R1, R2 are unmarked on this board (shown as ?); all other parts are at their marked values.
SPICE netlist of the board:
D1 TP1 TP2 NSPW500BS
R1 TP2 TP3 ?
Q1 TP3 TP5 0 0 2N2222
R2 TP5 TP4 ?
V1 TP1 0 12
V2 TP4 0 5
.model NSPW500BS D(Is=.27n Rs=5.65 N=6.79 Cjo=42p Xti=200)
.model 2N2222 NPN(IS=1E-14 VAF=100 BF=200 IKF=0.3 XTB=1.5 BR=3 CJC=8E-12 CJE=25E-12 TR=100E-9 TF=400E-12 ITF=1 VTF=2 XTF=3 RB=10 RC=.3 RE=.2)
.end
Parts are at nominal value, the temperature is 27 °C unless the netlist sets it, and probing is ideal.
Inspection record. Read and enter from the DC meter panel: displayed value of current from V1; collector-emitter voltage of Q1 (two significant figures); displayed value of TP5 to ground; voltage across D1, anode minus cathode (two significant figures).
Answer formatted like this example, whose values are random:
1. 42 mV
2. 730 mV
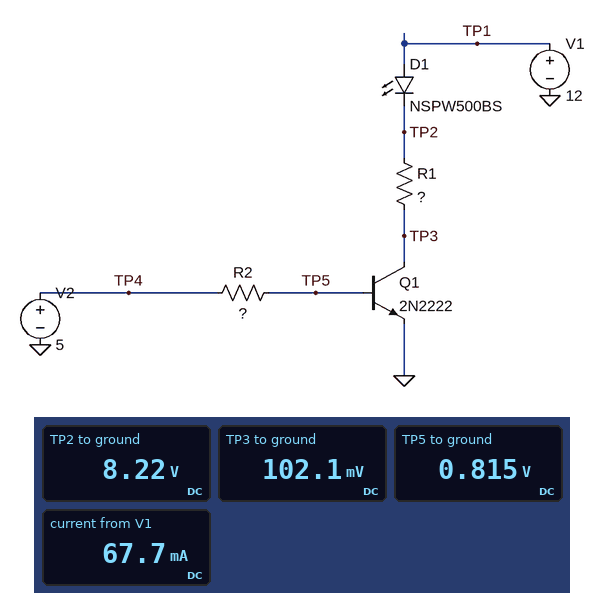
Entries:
1. 67.7 mA
2. 100 mV
3. 0.815 V
4. 3.8 V
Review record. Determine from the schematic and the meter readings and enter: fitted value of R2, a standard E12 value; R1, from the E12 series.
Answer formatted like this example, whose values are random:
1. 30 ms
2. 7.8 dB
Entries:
1. 1.5 kΩ
2. 120 Ω
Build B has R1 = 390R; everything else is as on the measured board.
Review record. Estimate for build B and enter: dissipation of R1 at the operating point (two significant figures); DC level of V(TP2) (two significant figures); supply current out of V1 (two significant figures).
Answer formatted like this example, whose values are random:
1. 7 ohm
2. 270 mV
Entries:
1. 190 mW
2. 8.7 V
3. 22 mA
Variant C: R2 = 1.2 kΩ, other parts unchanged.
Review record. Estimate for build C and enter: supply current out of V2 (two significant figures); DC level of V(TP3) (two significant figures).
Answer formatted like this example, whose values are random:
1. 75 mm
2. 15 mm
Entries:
1. 3.5 mA
2. 97 mV
